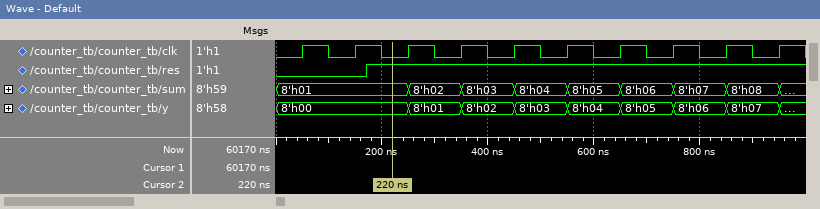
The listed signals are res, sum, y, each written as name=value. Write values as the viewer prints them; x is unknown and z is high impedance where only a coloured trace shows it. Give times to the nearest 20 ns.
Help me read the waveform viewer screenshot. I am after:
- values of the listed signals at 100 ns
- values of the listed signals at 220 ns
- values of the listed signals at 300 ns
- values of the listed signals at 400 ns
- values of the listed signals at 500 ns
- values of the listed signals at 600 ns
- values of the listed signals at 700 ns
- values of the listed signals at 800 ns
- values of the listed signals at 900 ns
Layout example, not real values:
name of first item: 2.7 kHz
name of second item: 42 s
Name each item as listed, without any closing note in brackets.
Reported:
values of the listed signals at 100 ns: res=0, sum=8'h01, y=8'h00
values of the listed signals at 220 ns: res=1, sum=8'h01, y=8'h00
values of the listed signals at 300 ns: res=1, sum=8'h02, y=8'h01
values of the listed signals at 400 ns: res=1, sum=8'h03, y=8'h02
values of the listed signals at 500 ns: res=1, sum=8'h04, y=8'h03
values of the listed signals at 600 ns: res=1, sum=8'h05, y=8'h04
values of the listed signals at 700 ns: res=1, sum=8'h06, y=8'h05
values of the listed signals at 800 ns: res=1, sum=8'h07, y=8'h06
values of the listed signals at 900 ns: res=1, sum=8'h08, y=8'h07
